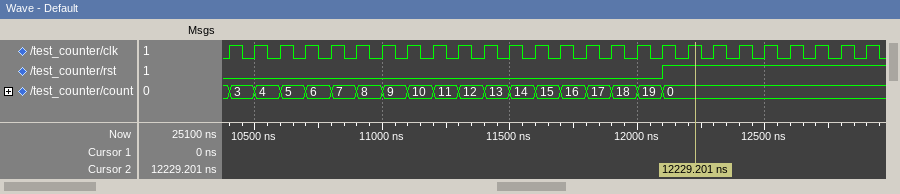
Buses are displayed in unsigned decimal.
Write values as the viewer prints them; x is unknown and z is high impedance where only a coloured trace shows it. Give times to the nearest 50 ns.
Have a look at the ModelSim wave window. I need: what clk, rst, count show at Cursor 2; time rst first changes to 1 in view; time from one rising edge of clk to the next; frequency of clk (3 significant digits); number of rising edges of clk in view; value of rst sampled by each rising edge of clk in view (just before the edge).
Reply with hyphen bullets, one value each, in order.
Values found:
- clk=1, rst=1, count=0
- 12100 ns
- 100 ns
- 10.0 MHz
- 26
- 0 0 0 0 0 0 0 0 0 0 0 0 0 0 0 0 0 0 1 1 1 1 1 1 1 1
